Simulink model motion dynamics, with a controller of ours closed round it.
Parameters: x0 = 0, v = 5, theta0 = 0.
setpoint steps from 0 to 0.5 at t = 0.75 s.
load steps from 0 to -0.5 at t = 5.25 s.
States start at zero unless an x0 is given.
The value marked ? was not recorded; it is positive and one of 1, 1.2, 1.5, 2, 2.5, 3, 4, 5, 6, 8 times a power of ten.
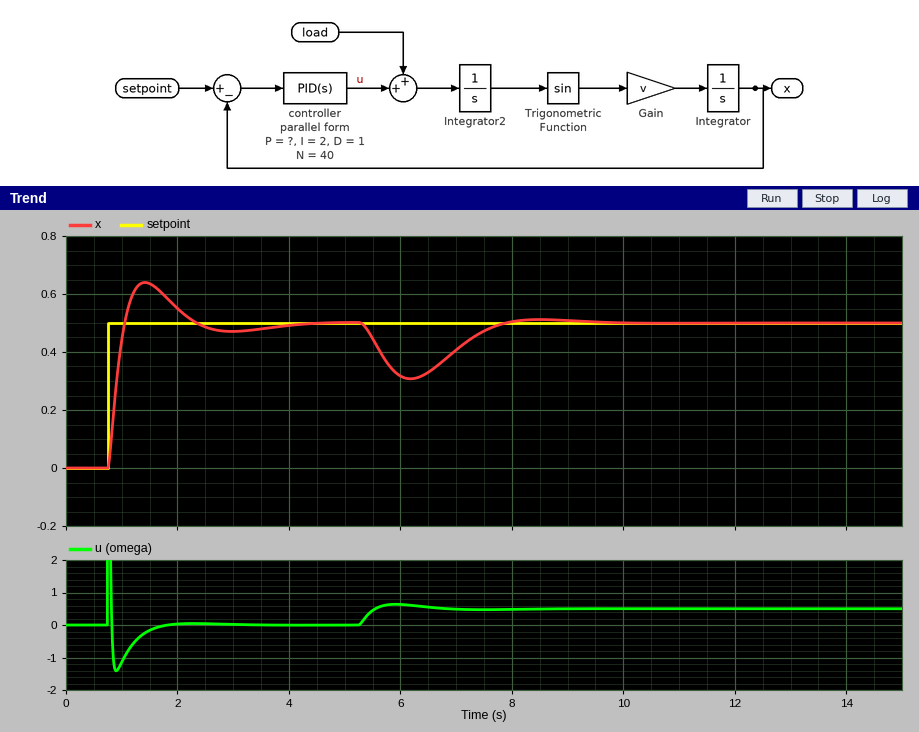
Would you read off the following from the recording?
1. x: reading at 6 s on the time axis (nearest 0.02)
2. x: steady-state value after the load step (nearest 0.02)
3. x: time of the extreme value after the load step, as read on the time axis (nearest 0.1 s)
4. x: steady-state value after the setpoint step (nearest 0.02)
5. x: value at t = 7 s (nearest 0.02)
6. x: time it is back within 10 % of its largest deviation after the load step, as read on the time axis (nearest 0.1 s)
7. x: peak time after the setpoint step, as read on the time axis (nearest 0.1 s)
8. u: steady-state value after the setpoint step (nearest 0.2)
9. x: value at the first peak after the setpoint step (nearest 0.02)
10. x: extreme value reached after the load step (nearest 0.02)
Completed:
0.32
0.50
6.2 s
0.50
0.40
7.6 s
1.4 s
0.0
0.64
0.30
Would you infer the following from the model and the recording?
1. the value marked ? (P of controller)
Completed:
2
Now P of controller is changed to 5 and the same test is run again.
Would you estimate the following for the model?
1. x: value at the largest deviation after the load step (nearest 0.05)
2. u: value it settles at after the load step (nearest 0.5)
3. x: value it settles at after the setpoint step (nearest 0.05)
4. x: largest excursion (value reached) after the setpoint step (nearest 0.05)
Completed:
0.40
0.5
0.50
0.70
